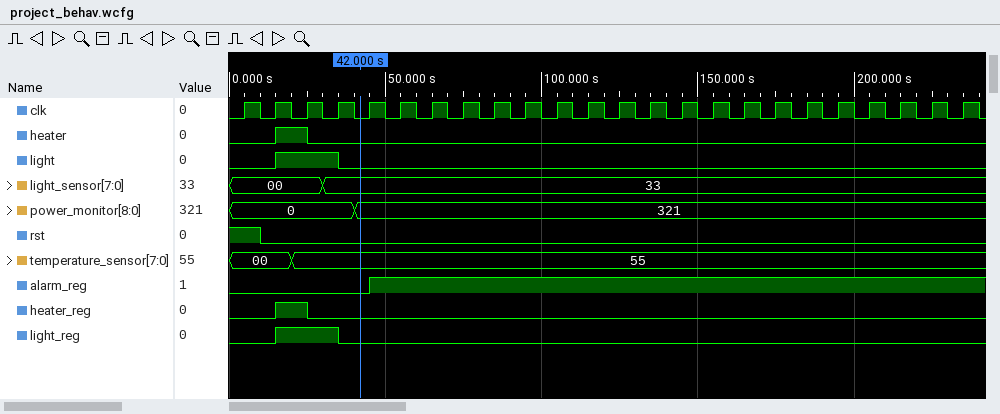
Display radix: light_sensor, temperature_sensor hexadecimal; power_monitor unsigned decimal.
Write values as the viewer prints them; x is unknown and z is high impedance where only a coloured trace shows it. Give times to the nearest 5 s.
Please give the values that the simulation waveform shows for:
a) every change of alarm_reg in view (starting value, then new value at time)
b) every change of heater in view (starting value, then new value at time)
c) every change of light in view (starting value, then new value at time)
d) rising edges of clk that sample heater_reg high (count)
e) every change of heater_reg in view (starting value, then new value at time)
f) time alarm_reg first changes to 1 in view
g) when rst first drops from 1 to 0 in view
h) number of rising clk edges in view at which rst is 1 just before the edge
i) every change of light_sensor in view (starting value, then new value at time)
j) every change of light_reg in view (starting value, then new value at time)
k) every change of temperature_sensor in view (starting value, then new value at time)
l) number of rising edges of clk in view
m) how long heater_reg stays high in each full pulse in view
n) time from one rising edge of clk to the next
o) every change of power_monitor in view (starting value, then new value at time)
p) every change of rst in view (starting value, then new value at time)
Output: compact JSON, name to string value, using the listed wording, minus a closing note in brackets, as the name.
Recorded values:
{"every change of alarm_reg in view": "0, 1 at 45 s", "every change of heater in view": "0, 1 at 15 s, 0 at 25 s", "every change of light in view": "0, 1 at 15 s, 0 at 35 s", "rising edges of clk that sample heater_reg high": "1", "every change of heater_reg in view": "0, 1 at 15 s, 0 at 25 s", "time alarm_reg first changes to 1 in view": "45 s", "when rst first drops from 1 to 0 in view": "10 s", "number of rising clk edges in view at which rst is 1 just before the edge": "1", "every change of light_sensor in view": "00, 33 at 30 s", "every change of light_reg in view": "0, 1 at 15 s, 0 at 35 s", "every change of temperature_sensor in view": "00, 55 at 20 s", "number of rising edges of clk in view": "24", "how long heater_reg stays high in each full pulse in view": "10 s", "time from one rising edge of clk to the next": "10 s", "every change of power_monitor in view": "0, 321 at 40 s", "every change of rst in view": "1, 0 at 10 s"}
